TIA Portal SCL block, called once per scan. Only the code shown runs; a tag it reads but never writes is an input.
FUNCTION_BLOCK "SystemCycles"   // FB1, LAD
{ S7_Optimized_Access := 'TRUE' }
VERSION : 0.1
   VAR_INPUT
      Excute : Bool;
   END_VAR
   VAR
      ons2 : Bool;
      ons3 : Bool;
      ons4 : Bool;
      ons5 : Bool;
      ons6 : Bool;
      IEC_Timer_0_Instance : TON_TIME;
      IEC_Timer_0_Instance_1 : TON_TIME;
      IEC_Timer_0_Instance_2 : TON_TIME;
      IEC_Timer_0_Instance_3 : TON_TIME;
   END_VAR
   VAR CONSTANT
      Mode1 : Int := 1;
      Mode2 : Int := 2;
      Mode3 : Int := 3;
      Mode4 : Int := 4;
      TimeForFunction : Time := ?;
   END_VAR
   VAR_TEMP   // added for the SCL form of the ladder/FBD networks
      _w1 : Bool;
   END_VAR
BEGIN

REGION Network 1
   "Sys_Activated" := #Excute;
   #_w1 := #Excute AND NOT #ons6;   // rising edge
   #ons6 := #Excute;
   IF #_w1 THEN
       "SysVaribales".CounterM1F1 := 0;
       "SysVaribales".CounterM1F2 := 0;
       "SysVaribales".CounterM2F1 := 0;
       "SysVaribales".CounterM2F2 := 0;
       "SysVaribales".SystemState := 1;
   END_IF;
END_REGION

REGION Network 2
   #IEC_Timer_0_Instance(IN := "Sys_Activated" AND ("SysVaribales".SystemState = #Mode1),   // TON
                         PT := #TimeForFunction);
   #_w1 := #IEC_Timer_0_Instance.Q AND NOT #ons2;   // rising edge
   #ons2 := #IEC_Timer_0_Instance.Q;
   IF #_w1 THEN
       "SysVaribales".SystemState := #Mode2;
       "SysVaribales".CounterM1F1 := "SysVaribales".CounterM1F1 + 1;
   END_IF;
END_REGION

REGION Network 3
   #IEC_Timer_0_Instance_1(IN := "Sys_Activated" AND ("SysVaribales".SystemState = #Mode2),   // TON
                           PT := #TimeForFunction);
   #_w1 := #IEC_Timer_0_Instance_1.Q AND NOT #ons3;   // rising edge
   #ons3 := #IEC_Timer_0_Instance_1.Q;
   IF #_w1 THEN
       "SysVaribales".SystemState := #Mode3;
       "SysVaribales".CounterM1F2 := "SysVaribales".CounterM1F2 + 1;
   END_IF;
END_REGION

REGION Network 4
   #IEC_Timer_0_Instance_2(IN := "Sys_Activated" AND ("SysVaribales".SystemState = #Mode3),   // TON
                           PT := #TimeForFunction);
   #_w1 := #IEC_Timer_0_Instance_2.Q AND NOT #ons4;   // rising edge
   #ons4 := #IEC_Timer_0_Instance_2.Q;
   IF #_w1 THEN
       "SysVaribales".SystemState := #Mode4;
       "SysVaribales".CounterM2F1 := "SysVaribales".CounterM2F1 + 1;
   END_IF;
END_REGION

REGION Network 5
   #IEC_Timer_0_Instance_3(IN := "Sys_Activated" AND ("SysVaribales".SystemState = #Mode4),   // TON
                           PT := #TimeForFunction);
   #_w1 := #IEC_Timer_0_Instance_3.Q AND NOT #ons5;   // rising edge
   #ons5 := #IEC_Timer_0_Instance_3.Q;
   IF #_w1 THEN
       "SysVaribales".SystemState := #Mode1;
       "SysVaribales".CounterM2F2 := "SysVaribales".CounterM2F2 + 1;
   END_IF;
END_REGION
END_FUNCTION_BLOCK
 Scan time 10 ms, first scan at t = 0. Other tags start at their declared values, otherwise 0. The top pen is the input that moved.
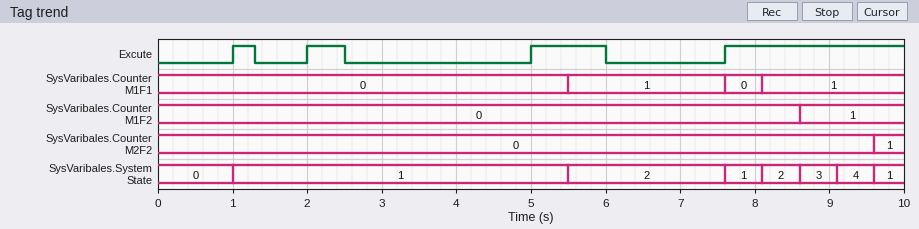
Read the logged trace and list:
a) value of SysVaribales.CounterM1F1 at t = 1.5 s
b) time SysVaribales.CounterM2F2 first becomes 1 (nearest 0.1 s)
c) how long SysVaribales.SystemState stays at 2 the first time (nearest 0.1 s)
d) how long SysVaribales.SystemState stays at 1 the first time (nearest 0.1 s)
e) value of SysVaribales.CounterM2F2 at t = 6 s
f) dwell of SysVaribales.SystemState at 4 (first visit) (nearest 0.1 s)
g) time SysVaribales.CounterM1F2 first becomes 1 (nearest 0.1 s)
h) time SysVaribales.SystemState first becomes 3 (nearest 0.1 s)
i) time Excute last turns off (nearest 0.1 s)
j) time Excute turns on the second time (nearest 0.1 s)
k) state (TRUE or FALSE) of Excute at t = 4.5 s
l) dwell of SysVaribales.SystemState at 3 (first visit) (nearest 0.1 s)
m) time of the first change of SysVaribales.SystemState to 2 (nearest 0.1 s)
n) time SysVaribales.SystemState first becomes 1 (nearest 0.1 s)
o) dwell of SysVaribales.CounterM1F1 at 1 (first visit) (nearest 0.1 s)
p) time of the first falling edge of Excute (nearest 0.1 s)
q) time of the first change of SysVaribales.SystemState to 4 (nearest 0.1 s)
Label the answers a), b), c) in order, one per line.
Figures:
a) 0
b) 9.6 s
c) 2.1 s
d) 4.5 s
e) 0
f) 0.5 s
g) 8.6 s
h) 8.6 s
i) 6.0 s
j) 2.0 s
k) FALSE
l) 0.5 s
m) 5.5 s
n) 1.0 s
o) 2.1 s
p) 1.3 s
q) 9.1 s
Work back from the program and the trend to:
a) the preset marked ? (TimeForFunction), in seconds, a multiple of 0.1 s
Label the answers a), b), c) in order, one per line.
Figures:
a) 0.5 s
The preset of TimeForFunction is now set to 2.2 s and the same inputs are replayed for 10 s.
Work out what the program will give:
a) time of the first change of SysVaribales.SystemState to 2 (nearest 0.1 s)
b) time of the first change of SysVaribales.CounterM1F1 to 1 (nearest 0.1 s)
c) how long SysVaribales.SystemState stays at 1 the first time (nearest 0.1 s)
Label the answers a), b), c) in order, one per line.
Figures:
a) 9.8 s
b) 9.8 s
c) 8.8 s
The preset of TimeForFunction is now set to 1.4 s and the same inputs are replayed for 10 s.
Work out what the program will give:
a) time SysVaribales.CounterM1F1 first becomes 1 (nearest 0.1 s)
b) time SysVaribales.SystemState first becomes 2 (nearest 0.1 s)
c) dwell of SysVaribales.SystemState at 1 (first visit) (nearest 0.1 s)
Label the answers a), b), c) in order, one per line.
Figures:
a) 9.0 s
b) 9.0 s
c) 8.0 s
